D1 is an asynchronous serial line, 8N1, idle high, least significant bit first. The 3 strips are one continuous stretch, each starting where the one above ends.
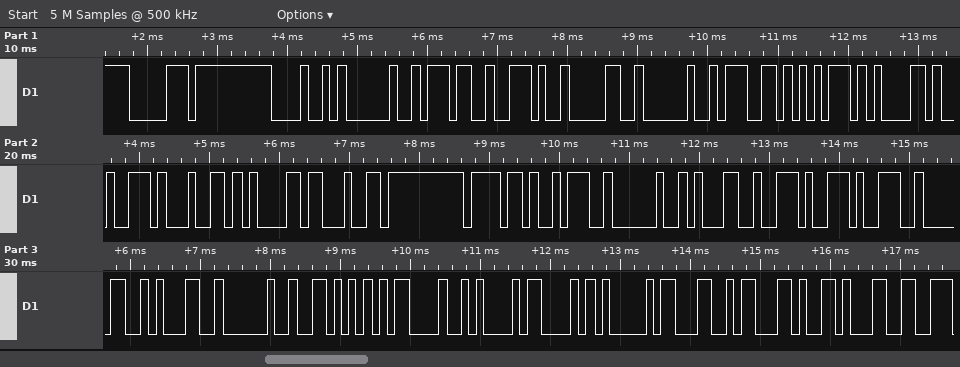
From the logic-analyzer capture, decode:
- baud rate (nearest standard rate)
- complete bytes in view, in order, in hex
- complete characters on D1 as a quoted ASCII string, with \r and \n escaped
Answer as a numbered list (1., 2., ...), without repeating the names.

1. 9600 baud
2. 0x70 0x48 0x20 0x37 0x2E 0x30 0x20 0x67 0x75 0x61 0x72 0x64 0x61 0x64 0x6F 0x3A 0x20 0x31 0x2E 0x39 0x30 0x31 0x20 0x56 0x0D 0x0A 0x43 0x41 0x4C 0x2C 0x31
3. "pH 7.0 guardado: 1.901 V\r\nCAL,1"
